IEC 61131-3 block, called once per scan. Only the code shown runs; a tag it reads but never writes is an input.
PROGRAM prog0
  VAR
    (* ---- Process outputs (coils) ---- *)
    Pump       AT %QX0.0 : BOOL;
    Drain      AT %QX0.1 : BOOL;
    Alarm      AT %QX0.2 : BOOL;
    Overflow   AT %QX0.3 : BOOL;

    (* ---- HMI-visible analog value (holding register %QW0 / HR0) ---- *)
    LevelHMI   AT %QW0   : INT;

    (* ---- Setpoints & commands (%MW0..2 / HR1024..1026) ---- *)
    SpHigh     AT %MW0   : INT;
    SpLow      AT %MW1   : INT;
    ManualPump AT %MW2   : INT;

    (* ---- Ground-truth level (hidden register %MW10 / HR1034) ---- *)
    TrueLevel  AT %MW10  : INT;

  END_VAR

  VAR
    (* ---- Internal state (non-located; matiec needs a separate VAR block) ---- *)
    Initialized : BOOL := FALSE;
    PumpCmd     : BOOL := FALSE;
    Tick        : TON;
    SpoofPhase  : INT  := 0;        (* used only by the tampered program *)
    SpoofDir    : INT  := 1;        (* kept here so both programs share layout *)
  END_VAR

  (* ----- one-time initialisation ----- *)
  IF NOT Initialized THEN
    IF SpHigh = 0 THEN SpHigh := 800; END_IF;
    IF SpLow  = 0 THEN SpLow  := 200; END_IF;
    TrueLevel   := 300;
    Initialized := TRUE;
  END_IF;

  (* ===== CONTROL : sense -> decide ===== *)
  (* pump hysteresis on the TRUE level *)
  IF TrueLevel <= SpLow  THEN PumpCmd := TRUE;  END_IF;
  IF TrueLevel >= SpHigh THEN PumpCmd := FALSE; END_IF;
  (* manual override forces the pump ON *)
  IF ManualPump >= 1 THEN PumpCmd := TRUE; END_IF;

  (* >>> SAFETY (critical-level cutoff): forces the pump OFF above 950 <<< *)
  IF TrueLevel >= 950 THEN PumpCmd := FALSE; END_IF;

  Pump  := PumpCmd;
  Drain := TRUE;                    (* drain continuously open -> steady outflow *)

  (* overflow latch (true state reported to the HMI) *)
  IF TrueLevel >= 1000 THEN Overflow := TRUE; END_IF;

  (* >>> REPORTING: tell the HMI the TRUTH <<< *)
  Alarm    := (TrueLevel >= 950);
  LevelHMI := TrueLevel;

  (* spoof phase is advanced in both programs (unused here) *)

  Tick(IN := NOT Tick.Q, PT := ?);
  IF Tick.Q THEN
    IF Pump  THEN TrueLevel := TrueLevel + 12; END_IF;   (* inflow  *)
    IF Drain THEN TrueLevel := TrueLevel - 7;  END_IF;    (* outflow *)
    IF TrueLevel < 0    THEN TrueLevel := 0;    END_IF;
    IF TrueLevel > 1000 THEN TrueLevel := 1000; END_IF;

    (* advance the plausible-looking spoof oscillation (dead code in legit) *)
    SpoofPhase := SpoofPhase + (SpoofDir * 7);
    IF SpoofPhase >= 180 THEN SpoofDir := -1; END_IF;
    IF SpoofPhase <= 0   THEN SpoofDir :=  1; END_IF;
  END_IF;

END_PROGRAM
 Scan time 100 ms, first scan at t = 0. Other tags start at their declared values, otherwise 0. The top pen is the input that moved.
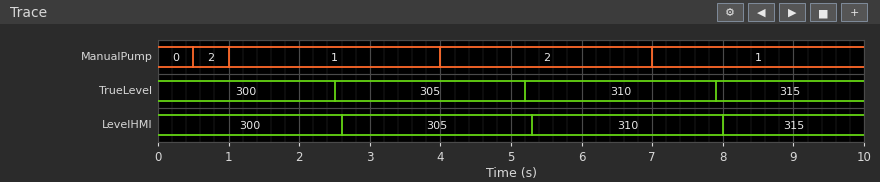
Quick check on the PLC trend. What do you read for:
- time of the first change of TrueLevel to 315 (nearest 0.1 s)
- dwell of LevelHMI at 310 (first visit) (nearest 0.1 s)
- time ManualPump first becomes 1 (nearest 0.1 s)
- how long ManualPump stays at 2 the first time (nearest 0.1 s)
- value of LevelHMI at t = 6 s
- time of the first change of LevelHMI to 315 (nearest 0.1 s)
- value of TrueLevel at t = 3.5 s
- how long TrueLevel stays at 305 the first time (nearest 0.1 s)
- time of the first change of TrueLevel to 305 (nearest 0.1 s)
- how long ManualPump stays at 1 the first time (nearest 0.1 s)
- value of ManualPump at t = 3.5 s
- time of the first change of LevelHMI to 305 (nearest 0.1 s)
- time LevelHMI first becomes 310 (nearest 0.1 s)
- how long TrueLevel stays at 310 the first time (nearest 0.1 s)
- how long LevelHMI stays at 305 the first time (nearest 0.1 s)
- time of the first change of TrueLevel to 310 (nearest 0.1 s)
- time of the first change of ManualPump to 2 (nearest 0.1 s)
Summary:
7.9 s
2.7 s
1.0 s
0.5 s
310
8.0 s
305
2.7 s
2.5 s
3.0 s
1
2.6 s
5.3 s
2.7 s
2.7 s
5.2 s
0.5 s
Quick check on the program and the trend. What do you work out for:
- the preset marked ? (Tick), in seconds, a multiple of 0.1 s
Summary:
2.5 s
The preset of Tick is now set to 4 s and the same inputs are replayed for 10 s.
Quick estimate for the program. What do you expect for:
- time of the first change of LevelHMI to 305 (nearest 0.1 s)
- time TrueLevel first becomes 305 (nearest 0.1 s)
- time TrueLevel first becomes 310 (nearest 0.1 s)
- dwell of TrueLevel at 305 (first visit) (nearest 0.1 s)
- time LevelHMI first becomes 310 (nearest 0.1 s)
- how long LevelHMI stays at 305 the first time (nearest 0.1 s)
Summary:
4.1 s
4.0 s
8.2 s
4.2 s
8.3 s
4.2 s
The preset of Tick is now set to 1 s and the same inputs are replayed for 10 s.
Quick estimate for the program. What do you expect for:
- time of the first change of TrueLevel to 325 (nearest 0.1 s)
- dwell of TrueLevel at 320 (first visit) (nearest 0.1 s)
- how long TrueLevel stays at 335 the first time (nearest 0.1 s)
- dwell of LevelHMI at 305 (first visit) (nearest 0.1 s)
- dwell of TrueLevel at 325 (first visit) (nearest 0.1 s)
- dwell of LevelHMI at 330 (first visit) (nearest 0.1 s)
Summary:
5.8 s
1.2 s
1.2 s
1.2 s
1.2 s
1.2 s
